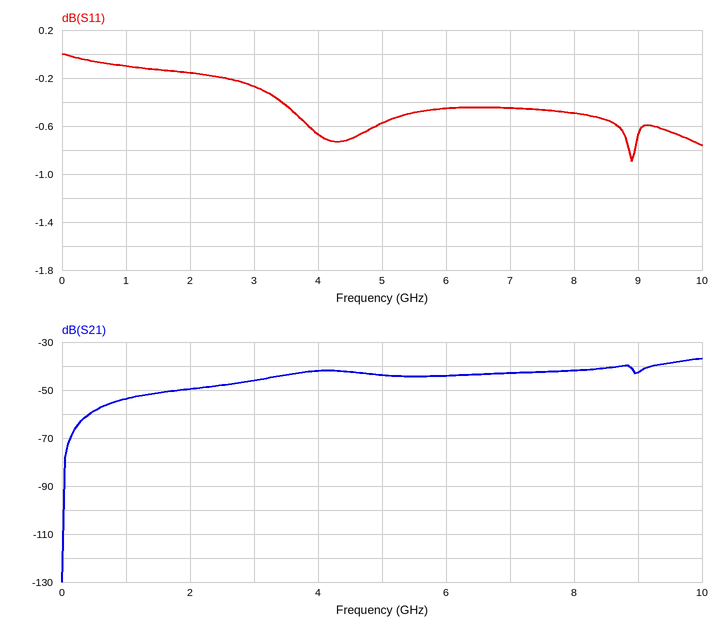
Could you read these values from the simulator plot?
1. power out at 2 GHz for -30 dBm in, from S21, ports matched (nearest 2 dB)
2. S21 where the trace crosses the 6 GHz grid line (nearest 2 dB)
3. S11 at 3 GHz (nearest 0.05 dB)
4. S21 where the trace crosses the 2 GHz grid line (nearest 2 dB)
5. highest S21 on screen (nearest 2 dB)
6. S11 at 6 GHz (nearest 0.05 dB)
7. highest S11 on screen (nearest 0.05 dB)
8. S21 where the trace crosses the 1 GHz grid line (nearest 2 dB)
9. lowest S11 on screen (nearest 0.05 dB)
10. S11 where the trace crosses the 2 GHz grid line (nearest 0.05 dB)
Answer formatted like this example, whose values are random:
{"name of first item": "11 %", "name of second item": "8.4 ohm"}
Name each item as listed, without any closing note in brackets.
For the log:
{"power out at 2 GHz for -30 dBm in, from S21, ports matched": "-80 dBm", "S21 where the trace crosses the 6 GHz grid line": "-44 dB", "S11 at 3 GHz": "-0.25 dB", "S21 where the trace crosses the 2 GHz grid line": "-50 dB", "highest S21 on screen": "-36 dB", "S11 at 6 GHz": "-0.45 dB", "highest S11 on screen": "0.00 dB", "S21 where the trace crosses the 1 GHz grid line": "-54 dB", "lowest S11 on screen": "-0.90 dB", "S11 where the trace crosses the 2 GHz grid line": "-0.15 dB"}
